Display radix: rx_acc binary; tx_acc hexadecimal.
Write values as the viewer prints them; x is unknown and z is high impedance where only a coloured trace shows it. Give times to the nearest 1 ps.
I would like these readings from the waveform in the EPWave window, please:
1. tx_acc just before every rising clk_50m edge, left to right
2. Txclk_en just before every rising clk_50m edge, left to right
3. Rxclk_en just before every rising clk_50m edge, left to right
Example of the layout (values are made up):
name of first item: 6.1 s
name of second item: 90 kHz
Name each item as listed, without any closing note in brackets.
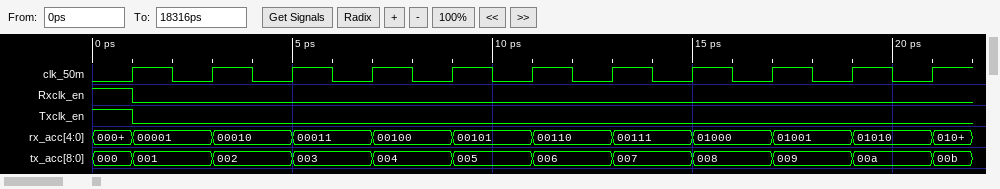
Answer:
tx_acc just before every rising clk_50m edge, left to right: 000, 001, 002, 003, 004, 005, 006, 007, 008, 009, 00a
Txclk_en just before every rising clk_50m edge, left to right: 1 0 0 0 0 0 0 0 0 0 0
Rxclk_en just before every rising clk_50m edge, left to right: 1 0 0 0 0 0 0 0 0 0 0
